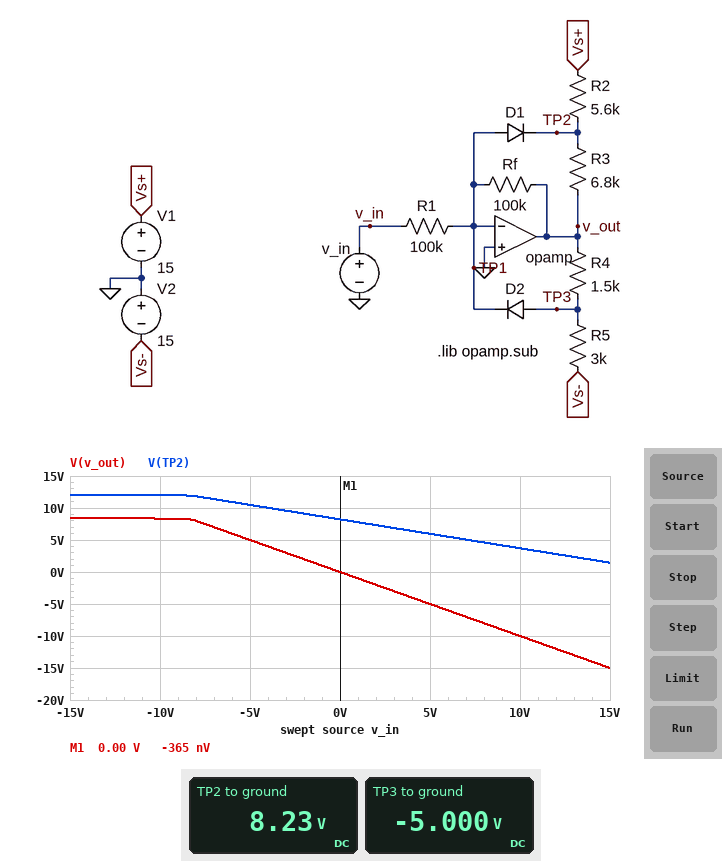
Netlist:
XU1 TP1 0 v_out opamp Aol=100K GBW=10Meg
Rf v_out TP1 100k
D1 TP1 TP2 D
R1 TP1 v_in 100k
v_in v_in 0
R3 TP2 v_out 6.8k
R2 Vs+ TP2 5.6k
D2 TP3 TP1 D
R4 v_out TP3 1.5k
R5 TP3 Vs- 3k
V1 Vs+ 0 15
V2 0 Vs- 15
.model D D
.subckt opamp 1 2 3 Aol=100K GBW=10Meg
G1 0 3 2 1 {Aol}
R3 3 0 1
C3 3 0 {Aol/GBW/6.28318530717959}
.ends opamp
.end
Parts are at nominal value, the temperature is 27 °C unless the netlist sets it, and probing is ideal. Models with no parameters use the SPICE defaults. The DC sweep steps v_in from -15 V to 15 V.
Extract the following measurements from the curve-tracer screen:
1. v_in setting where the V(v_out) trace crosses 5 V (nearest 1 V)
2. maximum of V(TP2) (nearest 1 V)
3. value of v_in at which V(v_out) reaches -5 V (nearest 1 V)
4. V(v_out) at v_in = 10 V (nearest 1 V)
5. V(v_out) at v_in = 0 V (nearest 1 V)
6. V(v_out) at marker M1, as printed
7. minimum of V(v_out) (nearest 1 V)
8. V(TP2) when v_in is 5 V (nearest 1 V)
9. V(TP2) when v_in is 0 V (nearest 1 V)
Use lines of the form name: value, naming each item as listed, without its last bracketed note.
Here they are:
v_in setting where the V(v_out) trace crosses 5 V: -5 V
maximum of V(TP2): 12 V
value of v_in at which V(v_out) reaches -5 V: 5 V
V(v_out) at v_in = 10 V: -10 V
V(v_out) at v_in = 0 V: 0 V
V(v_out) at marker M1, as printed: -365 nV
minimum of V(v_out): -15 V
V(TP2) when v_in is 5 V: 6 V
V(TP2) when v_in is 0 V: 8 V
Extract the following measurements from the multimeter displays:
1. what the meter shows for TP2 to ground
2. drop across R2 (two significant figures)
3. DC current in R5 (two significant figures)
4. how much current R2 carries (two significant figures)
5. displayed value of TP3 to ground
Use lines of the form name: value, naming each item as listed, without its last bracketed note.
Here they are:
what the meter shows for TP2 to ground: 8.23 V
drop across R2: 6.8 V
DC current in R5: 3.3 mA
how much current R2 carries: 1.2 mA
displayed value of TP3 to ground: -5.000 V
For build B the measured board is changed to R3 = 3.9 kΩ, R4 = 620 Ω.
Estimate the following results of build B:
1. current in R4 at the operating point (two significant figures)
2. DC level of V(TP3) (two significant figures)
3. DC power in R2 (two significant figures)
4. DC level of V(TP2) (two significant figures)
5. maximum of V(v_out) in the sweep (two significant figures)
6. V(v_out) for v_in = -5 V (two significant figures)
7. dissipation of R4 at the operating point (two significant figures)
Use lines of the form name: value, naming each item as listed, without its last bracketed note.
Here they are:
current in R4 at the operating point: 4.1 mA
DC level of V(TP3): -2.6 V
DC power in R2: 14 mW
DC level of V(TP2): 6.2 V
maximum of V(v_out) in the sweep: 3.9 V
V(v_out) for v_in = -5 V: 3.8 V
dissipation of R4 at the operating point: 11 mW
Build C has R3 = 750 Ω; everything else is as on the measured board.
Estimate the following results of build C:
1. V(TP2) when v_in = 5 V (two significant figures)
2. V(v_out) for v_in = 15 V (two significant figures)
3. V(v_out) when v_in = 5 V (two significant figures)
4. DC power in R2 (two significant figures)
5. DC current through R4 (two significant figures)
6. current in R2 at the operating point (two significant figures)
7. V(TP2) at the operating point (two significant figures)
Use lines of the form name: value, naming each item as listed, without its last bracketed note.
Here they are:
V(TP2) when v_in = 5 V: -560 mV
V(v_out) for v_in = 15 V: -2.8 V
V(v_out) when v_in = 5 V: -2.7 V
DC power in R2: 31 mW
DC current through R4: 3.3 mA
current in R2 at the operating point: 2.4 mA
V(TP2) at the operating point: 1.8 V
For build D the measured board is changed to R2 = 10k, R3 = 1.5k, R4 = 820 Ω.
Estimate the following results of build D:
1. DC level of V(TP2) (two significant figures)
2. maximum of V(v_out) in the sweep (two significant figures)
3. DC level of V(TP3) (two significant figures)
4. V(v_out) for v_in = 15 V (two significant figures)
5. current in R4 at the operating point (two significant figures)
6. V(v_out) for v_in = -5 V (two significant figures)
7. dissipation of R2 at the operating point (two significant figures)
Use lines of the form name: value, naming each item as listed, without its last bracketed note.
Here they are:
DC level of V(TP2): 2.0 V
maximum of V(v_out) in the sweep: 4.9 V
DC level of V(TP3): -3.2 V
V(v_out) for v_in = 15 V: -3.1 V
current in R4 at the operating point: 3.9 mA
V(v_out) for v_in = -5 V: 4.7 V
dissipation of R2 at the operating point: 17 mW
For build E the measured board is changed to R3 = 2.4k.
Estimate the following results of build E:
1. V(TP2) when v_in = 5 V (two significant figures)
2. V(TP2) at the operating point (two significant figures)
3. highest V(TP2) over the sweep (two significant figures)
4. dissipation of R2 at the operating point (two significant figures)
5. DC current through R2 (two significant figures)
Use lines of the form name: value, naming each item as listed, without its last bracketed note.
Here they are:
V(TP2) when v_in = 5 V: 1.0 V
V(TP2) at the operating point: 4.5 V
highest V(TP2) over the sweep: 10 V
dissipation of R2 at the operating point: 20 mW
DC current through R2: 1.9 mA
